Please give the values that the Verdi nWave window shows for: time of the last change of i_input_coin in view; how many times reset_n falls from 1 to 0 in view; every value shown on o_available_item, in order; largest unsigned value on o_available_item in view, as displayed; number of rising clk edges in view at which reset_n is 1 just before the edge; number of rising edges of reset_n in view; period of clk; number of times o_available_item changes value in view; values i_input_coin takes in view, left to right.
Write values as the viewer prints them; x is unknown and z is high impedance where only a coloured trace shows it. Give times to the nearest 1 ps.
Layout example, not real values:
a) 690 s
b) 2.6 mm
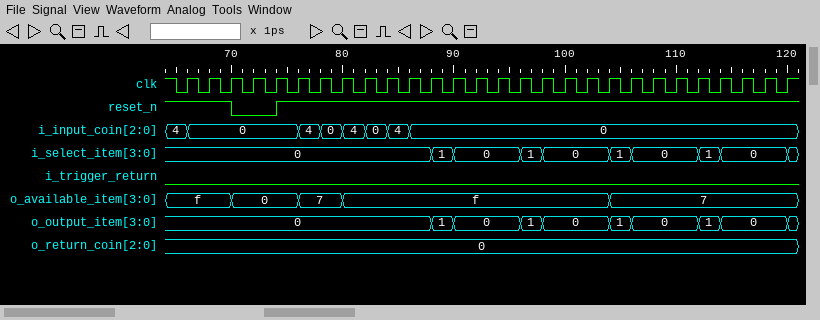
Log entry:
a) 86 ps
b) 1
c) f, 0, 7, f, 7
d) f
e) 26
f) 1
g) 2 ps
h) 4
i) 4, 0, 4, 0, 4, 0, 4, 0
